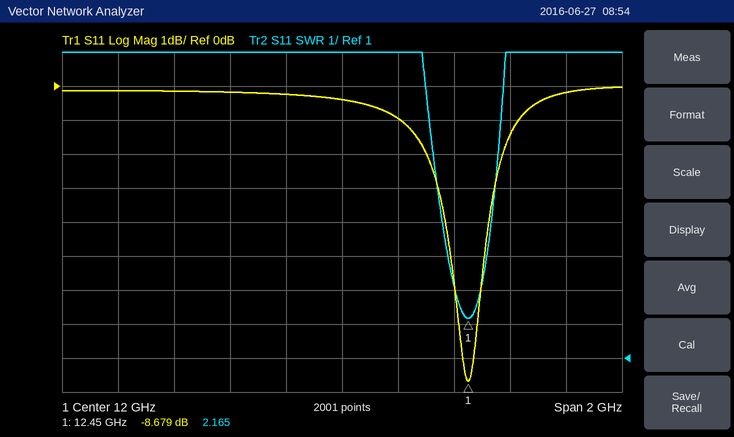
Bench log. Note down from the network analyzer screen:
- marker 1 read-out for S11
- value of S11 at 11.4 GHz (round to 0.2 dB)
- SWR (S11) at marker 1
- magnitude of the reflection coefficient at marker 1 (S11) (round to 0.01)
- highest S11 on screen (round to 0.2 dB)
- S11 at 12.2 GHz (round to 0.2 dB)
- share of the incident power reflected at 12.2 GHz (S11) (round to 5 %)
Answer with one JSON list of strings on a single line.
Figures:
["-8.679 dB", "-0.2 dB", "2.165", "0.37", "0.0 dB", "-1.0 dB", "80 %"]
